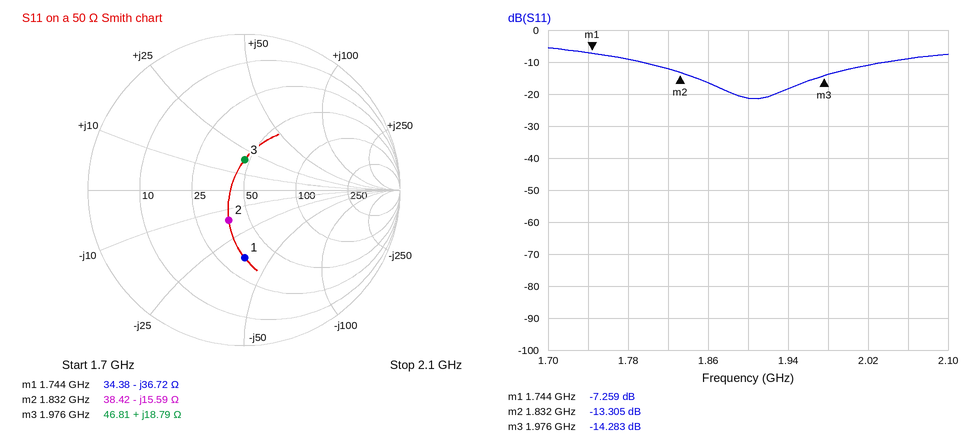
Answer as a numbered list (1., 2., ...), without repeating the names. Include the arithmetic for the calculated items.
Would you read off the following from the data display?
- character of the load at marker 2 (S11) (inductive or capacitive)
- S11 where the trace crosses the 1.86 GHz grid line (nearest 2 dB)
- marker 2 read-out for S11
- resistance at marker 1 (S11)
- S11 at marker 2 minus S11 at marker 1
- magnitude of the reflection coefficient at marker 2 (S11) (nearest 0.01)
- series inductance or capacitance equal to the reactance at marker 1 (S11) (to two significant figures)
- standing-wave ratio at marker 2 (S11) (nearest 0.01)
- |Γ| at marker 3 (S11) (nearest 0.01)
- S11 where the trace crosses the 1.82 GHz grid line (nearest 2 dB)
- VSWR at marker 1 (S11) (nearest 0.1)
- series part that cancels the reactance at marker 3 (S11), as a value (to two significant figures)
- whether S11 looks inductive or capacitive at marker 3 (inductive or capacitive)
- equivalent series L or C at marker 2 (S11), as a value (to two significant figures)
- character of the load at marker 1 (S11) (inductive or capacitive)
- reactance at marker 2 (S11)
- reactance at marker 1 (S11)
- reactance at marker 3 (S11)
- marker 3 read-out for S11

1. capacitive
2. -16 dB
3. -13.305 dB
4. 34.38 Ω
5. -13.305 − (-7.259) = -6.046 dB
6. 10^(-13.305/20) ≈ 0.22
7. C = 1/(2π × 1.744 GHz × 36.72 Ω) ≈ 2.5 pF
8. 1.55
9. 0.19
10. -12 dB
11. 2.5
12. C = 1/(2π × 1.976 GHz × 18.79 Ω) ≈ 4.3 pF
13. inductive
14. C = 1/(2π × 1.832 GHz × 15.59 Ω) ≈ 5.6 pF
15. capacitive
16. -15.59 Ω
17. -36.72 Ω
18. +18.79 Ω
19. -14.283 dB
